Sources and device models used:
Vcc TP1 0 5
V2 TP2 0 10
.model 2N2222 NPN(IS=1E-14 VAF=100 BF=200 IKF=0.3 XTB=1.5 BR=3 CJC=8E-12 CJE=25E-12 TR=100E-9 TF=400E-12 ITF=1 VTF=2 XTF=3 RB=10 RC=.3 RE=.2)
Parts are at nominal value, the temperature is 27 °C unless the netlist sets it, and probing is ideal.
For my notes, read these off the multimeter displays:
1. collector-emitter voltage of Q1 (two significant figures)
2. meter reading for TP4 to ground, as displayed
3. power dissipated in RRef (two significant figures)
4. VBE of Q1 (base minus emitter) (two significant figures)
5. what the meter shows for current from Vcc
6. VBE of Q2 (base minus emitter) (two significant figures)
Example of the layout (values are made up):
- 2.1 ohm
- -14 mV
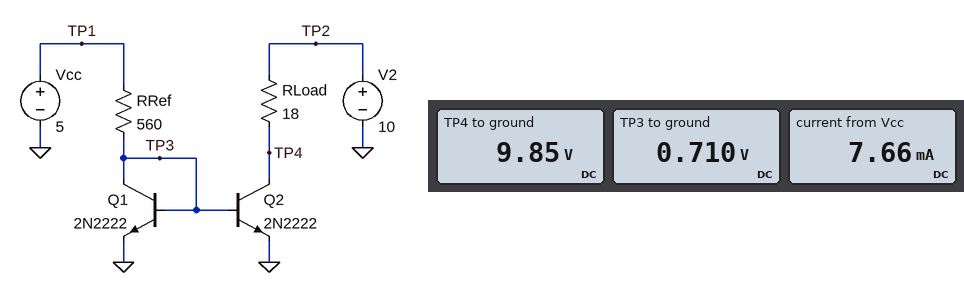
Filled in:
- 710 mV
- 9.85 V
- 33 mW
- 710 mV
- 7.66 mA
- 710 mV
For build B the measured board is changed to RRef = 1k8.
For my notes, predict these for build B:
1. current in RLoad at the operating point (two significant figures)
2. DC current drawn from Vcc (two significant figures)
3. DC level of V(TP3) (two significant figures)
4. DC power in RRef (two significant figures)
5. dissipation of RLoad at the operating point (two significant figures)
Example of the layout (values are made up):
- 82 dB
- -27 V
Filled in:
- 2.6 mA
- 2.4 mA
- 680 mV
- 10 mW
- 120 µW
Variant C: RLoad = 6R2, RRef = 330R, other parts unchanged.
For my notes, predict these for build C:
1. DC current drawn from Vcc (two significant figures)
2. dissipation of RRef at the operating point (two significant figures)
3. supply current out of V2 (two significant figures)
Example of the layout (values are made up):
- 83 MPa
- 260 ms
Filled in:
- 13 mA
- 55 mW
- 14 mA
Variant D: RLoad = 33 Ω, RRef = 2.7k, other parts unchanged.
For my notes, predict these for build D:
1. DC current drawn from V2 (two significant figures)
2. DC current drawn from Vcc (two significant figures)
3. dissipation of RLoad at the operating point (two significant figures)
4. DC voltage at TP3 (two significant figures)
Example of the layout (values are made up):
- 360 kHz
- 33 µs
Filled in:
- 1.7 mA
- 1.6 mA
- 99 µW
- 670 mV
